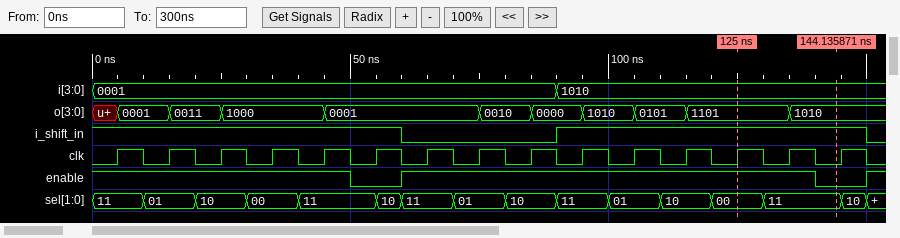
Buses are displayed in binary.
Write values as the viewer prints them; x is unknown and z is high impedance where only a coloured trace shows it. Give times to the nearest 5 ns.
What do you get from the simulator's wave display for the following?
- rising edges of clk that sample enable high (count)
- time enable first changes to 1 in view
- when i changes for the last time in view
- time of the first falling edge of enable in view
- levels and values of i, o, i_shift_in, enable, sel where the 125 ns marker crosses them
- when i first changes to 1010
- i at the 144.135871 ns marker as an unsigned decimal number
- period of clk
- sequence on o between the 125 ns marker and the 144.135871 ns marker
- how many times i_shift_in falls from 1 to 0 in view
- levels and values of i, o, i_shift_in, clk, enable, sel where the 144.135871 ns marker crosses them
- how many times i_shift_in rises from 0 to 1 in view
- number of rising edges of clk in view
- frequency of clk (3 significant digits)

13
60 ns
90 ns
50 ns
i=1010, o=1101, i_shift_in=1, enable=1, sel=00
90 ns
10
10 ns
1101, 1010
2
i=1010, o=1010, i_shift_in=1, clk=0, enable=0, sel=11
1
15
100 MHz
